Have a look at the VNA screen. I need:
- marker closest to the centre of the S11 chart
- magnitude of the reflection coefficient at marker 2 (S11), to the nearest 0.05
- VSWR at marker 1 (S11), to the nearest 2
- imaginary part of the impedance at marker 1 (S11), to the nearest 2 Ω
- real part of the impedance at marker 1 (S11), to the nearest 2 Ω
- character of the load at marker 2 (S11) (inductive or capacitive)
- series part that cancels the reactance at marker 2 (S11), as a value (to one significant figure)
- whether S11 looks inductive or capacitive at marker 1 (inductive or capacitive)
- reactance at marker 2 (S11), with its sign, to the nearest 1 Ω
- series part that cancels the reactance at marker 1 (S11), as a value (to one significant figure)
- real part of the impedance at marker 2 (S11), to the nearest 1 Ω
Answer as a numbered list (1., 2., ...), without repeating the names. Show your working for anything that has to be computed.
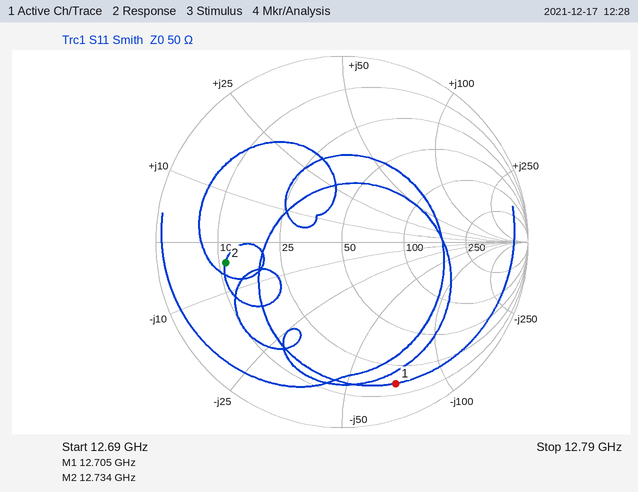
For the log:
1. marker 2
2. 0.65
3. 10
4. -70 Ω
5. 16 Ω
6. capacitive
7. L = 4 Ω/(2π × 12.734 GHz) ≈ 50 pH
8. capacitive
9. -4 Ω
10. L = 70 Ω/(2π × 12.705 GHz) ≈ 877 pH, so 900 pH to one significant figure
11. 11 Ω
